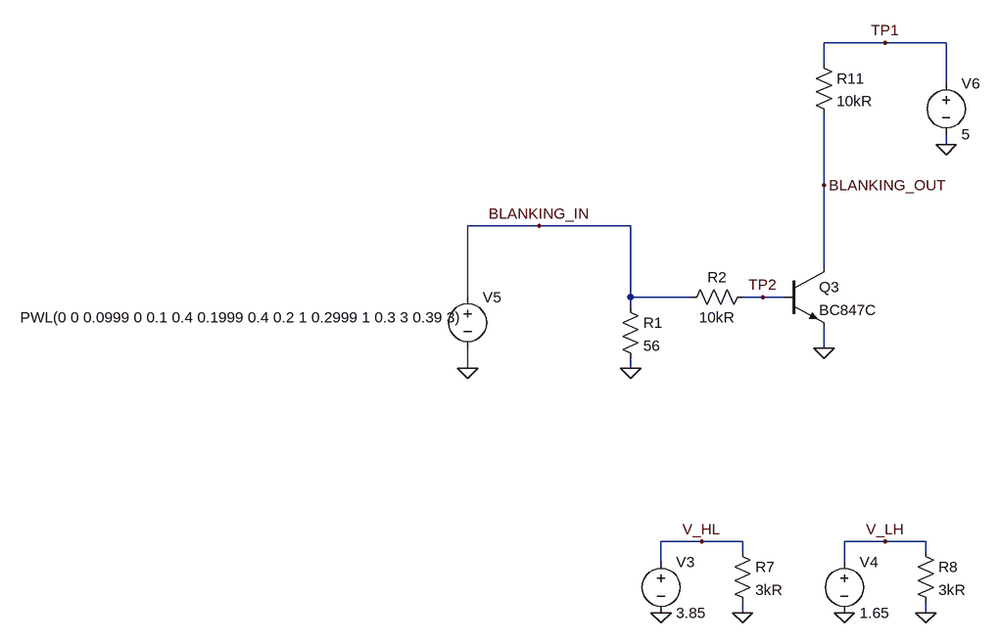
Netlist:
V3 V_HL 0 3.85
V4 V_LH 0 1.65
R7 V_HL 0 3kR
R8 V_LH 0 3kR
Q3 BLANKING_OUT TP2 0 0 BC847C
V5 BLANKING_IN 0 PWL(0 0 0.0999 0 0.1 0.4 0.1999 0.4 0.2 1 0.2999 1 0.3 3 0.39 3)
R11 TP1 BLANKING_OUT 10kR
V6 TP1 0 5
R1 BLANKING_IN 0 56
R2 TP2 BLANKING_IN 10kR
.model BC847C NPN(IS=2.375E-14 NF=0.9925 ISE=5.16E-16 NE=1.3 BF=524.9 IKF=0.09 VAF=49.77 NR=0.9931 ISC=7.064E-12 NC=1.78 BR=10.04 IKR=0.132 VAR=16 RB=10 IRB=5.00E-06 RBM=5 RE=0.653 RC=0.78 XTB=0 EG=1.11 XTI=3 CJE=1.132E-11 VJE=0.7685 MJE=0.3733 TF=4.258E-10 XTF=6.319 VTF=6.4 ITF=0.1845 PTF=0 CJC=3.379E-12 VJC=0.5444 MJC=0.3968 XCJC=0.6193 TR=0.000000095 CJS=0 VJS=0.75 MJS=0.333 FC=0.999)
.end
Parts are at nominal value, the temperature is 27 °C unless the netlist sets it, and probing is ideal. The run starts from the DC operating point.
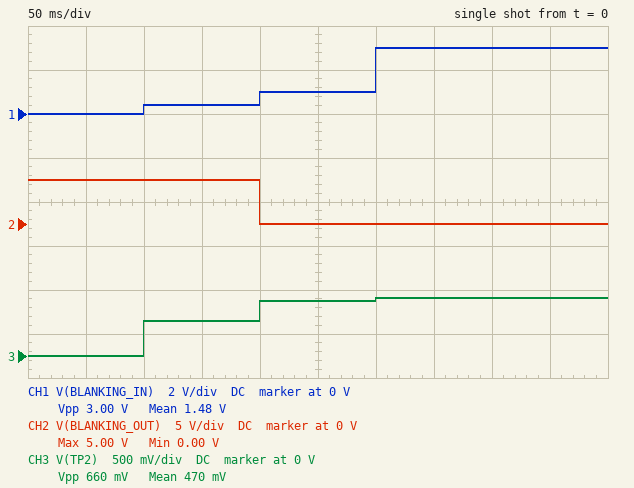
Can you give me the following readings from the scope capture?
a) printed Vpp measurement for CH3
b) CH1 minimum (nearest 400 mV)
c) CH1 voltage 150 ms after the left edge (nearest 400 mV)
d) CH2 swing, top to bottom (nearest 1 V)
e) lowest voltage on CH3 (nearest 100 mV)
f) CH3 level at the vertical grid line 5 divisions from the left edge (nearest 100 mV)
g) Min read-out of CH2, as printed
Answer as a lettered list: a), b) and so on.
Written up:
a) 660 mV
b) 0 V
c) 400 mV
d) 5 V
e) 0 V
f) 600 mV
g) 0.00 V
